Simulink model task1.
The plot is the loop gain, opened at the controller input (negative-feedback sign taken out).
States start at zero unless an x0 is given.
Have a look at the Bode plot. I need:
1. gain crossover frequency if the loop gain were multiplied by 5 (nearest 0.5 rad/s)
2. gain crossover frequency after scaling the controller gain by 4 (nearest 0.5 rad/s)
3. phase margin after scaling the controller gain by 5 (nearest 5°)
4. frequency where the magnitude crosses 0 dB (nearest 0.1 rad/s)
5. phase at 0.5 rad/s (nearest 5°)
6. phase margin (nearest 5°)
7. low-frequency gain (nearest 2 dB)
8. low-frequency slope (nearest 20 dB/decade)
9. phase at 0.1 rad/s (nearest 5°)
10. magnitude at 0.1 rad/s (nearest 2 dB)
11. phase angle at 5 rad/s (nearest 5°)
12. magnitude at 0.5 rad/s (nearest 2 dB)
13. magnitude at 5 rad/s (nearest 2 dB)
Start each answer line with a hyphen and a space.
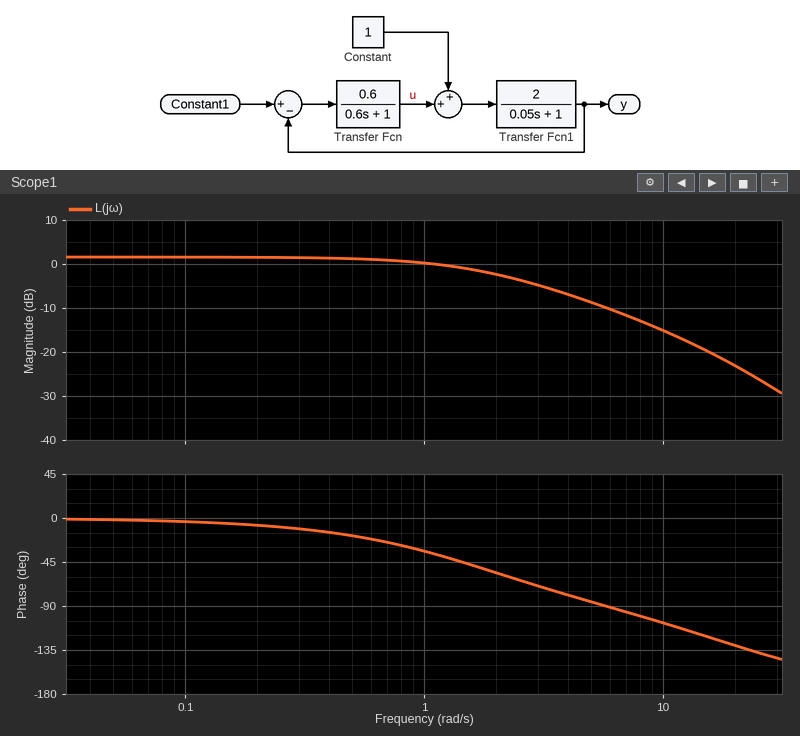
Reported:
- 9.0 rad/s
- 7.5 rad/s
- 75°
- 1.1 rad/s
- -20°
- 145°
- 2 dB
- 0 dB/decade
- -5°
- 2 dB
- -85°
- 2 dB
- -8 dB
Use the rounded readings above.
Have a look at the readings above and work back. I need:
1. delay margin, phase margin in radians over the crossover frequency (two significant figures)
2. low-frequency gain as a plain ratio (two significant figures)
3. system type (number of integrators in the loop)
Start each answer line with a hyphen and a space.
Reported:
- 2.3 s
- 1.3
- 0
